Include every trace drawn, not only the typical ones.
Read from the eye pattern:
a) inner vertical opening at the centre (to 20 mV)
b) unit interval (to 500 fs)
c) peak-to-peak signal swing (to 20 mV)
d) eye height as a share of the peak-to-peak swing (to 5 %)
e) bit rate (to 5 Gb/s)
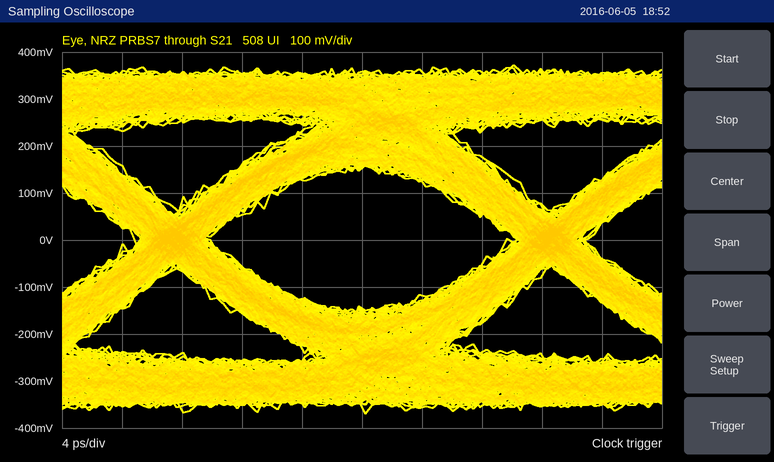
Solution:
300 mV
25.0 ps
740 mV
40 %
40 Gb/s
